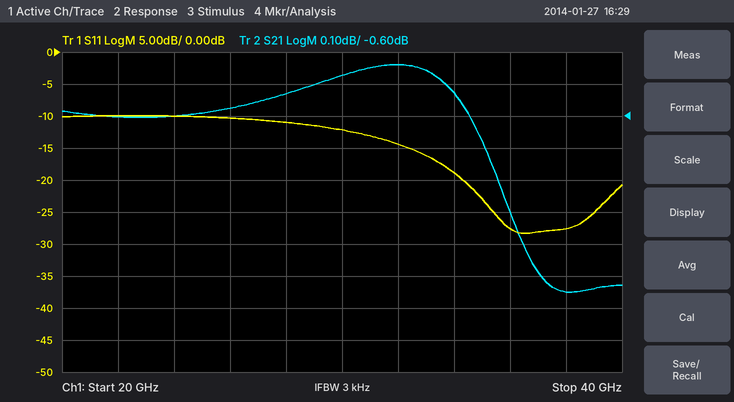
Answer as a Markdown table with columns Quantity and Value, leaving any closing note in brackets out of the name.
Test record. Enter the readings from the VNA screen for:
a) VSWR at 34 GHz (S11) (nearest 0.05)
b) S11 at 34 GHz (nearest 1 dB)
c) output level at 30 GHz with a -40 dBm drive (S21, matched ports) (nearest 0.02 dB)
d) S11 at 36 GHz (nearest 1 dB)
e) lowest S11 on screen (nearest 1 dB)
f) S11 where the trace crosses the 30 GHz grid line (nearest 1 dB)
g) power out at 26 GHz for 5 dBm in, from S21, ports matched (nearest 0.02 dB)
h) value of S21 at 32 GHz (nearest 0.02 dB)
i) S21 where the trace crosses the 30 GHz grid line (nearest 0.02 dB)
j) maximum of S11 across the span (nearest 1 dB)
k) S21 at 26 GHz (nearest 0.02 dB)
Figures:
| Quantity | Value |
|---|---|
| VSWR at 34 GHz (S11) | 1.25 |
| S11 at 34 GHz | -19 dB |
| output level at 30 GHz with a -40 dBm drive (S21, matched ports) | -40.48 dBm |
| S11 at 36 GHz | -28 dB |
| lowest S11 on screen | -28 dB |
| S11 where the trace crosses the 30 GHz grid line | -12 dB |
| power out at 26 GHz for 5 dBm in, from S21, ports matched | 4.42 dBm |
| value of S21 at 32 GHz | -0.44 dB |
| S21 where the trace crosses the 30 GHz grid line | -0.48 dB |
| maximum of S11 across the span | -10 dB |
| S21 at 26 GHz | -0.58 dB |
